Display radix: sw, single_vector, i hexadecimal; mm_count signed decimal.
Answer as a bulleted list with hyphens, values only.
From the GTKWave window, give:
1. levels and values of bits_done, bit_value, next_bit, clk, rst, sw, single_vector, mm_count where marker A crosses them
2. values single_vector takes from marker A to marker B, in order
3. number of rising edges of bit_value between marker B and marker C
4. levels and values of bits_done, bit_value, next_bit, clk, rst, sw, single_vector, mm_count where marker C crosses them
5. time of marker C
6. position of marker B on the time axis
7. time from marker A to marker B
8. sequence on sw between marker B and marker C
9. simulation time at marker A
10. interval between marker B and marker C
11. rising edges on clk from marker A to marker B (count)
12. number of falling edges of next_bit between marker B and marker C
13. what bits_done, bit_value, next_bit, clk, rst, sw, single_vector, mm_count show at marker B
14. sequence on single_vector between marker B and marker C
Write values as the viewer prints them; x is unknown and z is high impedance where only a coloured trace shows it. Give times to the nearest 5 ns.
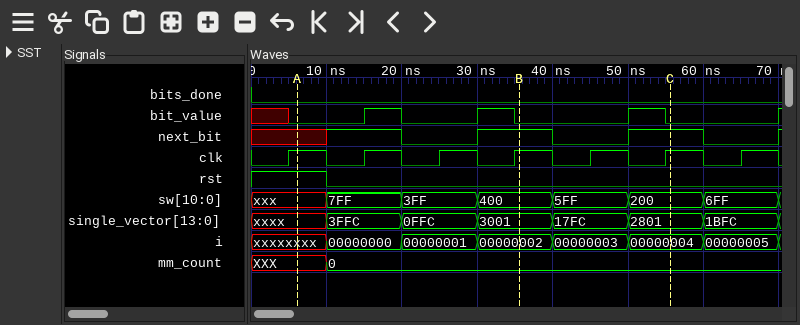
- bits_done=0, bit_value=0, next_bit=x, clk=1, rst=1, sw=xxx, single_vector=xxxx, mm_count=XXX
- xxxx, 3FFC, 0FFC, 3001
- 1
- bits_done=0, bit_value=0, next_bit=1, clk=1, rst=0, sw=200, single_vector=2801, mm_count=0
- 55 ns
- 35 ns
- 30 ns
- 400, 5FF, 200
- 5 ns
- 20 ns
- 3
- 1
- bits_done=0, bit_value=0, next_bit=1, clk=1, rst=0, sw=400, single_vector=3001, mm_count=0
- 3001, 17FC, 2801
